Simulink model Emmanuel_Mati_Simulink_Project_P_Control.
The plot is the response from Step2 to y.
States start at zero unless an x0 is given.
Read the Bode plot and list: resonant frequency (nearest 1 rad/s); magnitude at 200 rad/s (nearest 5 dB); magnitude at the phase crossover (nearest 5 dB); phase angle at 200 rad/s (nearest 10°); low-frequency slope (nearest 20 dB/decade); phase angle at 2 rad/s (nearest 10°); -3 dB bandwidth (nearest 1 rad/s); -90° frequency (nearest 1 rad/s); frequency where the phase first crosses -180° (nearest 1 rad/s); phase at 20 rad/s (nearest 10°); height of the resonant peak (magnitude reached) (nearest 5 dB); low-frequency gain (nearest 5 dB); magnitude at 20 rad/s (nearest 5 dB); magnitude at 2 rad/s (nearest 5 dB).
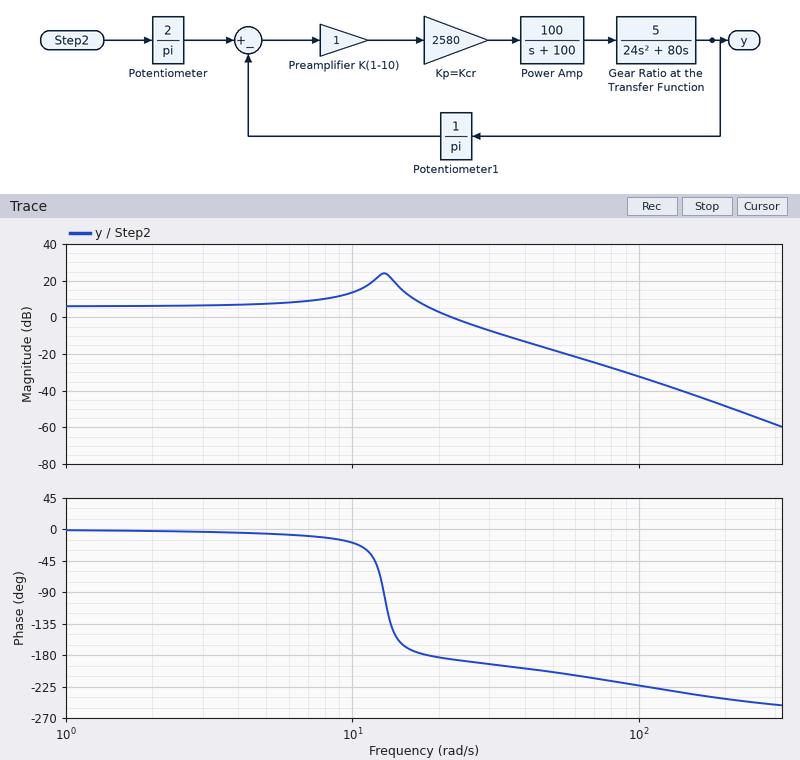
13 rad/s
-50 dB
5 dB
-240°
0 dB/decade
0°
20 rad/s
13 rad/s
18 rad/s
-180°
25 dB
5 dB
5 dB
5 dB
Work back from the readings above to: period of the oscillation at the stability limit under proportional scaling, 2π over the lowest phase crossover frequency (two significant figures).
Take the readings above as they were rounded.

0.35 s
